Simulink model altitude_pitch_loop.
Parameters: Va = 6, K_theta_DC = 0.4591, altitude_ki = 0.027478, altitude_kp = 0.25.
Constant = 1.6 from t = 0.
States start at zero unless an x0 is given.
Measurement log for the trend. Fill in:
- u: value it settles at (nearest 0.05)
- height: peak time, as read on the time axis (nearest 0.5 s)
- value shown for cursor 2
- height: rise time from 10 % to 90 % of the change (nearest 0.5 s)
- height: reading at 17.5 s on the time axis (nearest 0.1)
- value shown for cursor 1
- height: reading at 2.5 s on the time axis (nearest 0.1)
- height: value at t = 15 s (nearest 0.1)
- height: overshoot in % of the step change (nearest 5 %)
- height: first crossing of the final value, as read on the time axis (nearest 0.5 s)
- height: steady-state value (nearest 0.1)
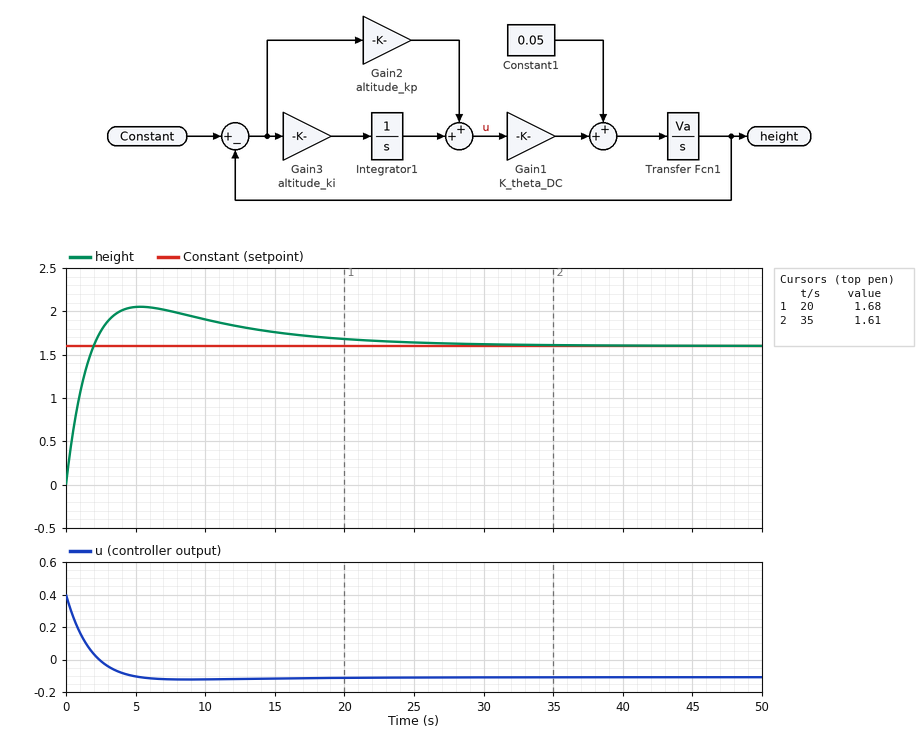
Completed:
-0.10
5.5 s
1.61
1.5 s
1.7
1.68
1.8
1.8
30 %
2.0 s
1.6
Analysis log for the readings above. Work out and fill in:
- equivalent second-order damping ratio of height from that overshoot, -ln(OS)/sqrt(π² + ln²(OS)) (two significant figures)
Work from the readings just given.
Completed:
0.36
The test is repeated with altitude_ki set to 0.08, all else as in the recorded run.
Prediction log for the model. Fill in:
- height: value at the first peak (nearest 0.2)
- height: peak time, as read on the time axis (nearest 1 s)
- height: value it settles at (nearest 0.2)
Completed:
2.2
4 s
1.6
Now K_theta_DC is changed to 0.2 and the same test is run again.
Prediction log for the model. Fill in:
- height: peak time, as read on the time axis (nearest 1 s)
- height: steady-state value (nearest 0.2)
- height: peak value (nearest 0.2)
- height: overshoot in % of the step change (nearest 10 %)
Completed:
9 s
1.6
2.4
50 %
